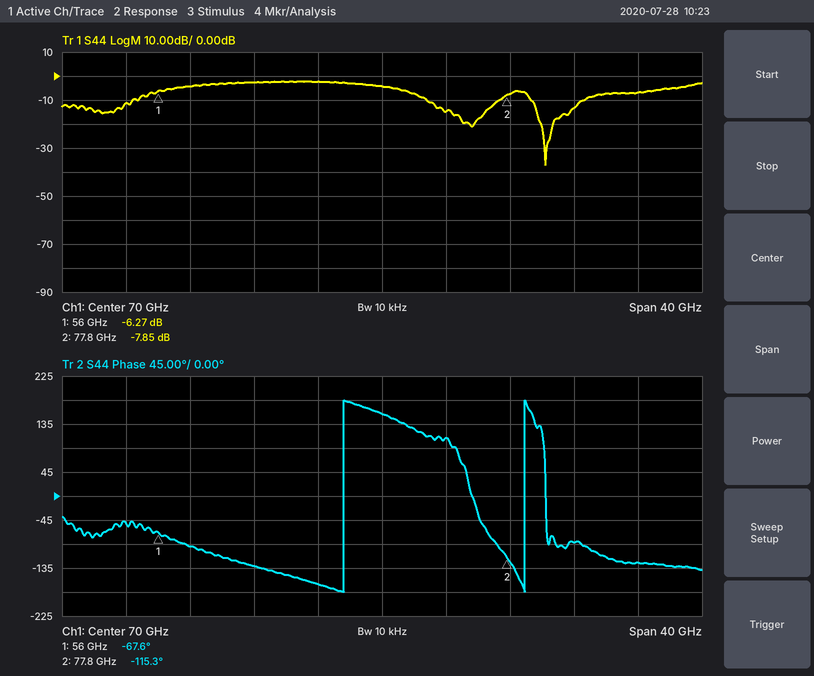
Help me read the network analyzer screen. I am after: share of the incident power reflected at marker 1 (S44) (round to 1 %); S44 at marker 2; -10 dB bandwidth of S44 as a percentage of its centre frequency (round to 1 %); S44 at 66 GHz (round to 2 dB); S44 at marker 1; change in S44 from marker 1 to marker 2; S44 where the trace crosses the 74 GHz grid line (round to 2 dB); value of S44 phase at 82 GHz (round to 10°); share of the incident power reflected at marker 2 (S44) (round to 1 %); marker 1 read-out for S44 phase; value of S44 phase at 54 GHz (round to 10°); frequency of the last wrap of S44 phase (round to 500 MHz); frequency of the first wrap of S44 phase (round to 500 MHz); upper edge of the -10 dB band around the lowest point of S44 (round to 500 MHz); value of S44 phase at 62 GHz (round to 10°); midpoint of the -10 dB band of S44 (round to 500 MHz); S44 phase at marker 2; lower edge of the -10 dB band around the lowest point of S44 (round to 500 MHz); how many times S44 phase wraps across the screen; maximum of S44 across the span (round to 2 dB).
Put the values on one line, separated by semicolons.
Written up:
24 %; -7.85 dB; 4 %; -2 dB; -6.27 dB; -1.58 dB; -14 dB; -90°; 16 %; -67.6°; -50°; 79.0 GHz; 67.5 GHz; 82.5 GHz; -130°; 81.0 GHz; -115.3°; 79.5 GHz; 2; -2 dB
